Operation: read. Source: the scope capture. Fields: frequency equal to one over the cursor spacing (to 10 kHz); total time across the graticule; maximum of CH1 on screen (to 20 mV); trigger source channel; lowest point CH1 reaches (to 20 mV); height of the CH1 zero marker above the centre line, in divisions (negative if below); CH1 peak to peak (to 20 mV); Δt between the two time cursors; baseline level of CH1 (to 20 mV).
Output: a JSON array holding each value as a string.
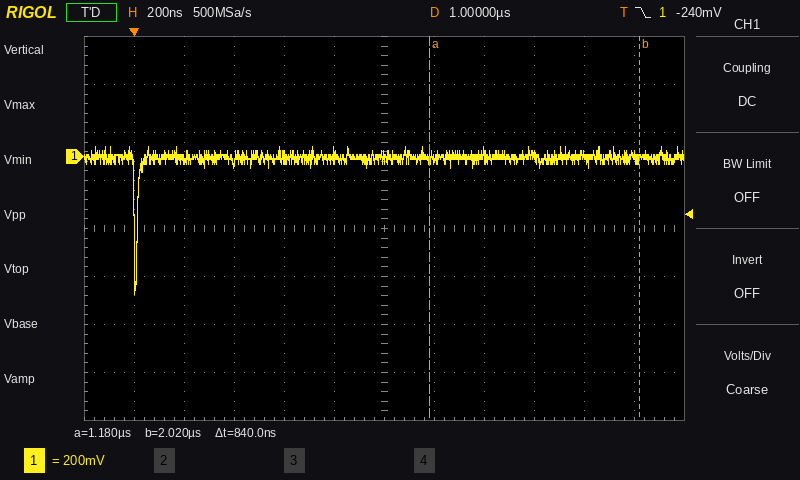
["1.19 MHz", "2.4 µs", "40 mV", "CH1", "-580 mV", "+1.5 div", "620 mV", "840 ns", "0 mV"]
